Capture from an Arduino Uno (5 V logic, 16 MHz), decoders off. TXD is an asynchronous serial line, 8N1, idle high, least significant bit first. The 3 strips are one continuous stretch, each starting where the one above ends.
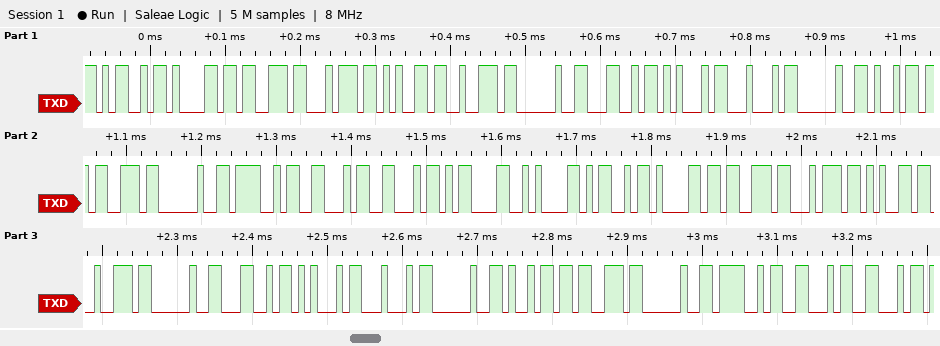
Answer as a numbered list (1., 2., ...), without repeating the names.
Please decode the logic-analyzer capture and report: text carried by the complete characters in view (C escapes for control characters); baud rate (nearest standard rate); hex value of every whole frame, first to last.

1. "Master LED is OFF\r\nMaster LED is OFF"
2. 115200 baud
3. 4D 61 73 74 65 72 20 4C 45 44 20 69 73 20 4F 46 46 0D 0A 4D 61 73 74 65 72 20 4C 45 44 20 69 73 20 4F 46 46
